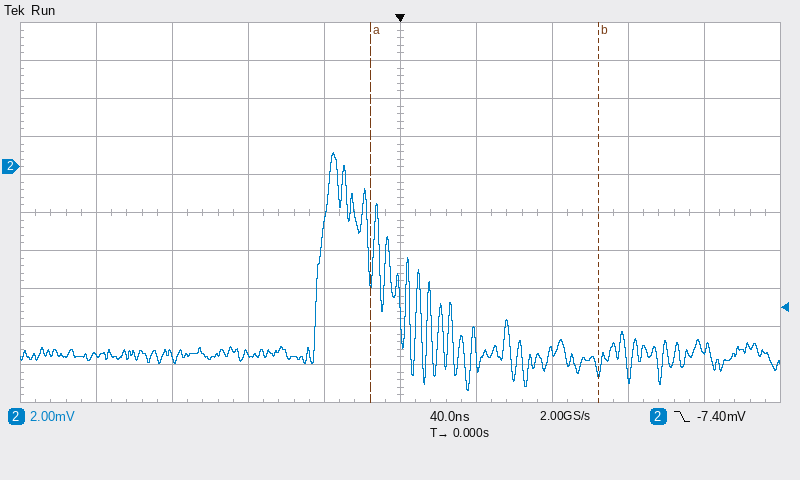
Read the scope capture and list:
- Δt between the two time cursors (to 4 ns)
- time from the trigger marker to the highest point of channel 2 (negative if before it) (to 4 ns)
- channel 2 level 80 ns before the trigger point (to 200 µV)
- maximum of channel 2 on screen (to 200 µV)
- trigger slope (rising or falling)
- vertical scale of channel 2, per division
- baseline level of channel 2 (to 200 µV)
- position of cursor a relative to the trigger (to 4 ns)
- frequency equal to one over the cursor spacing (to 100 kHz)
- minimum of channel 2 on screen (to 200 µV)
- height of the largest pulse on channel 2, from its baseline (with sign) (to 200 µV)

120 ns
-36 ns
-9.8 mV
800 µV
falling
2 mV
-9.8 mV
-16 ns
8.3 MHz
-11.8 mV
+10.6 mV
